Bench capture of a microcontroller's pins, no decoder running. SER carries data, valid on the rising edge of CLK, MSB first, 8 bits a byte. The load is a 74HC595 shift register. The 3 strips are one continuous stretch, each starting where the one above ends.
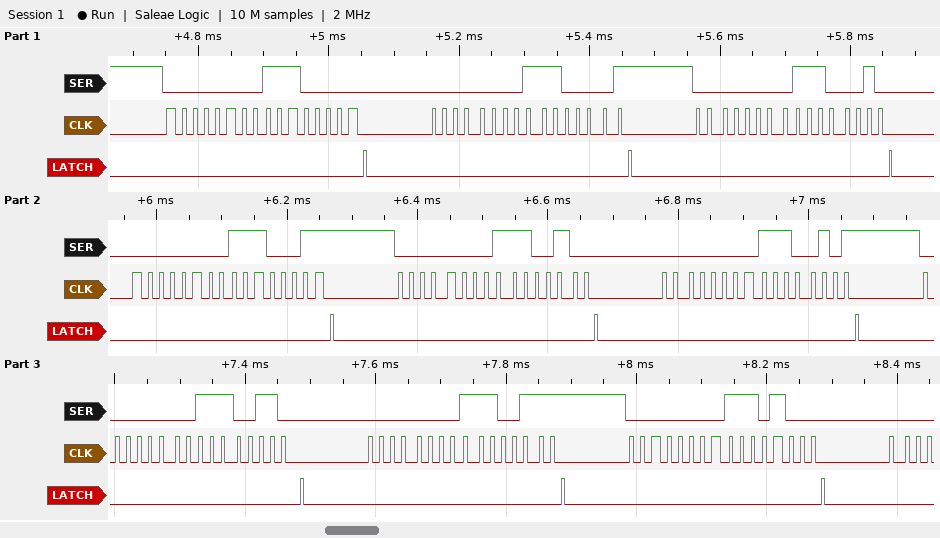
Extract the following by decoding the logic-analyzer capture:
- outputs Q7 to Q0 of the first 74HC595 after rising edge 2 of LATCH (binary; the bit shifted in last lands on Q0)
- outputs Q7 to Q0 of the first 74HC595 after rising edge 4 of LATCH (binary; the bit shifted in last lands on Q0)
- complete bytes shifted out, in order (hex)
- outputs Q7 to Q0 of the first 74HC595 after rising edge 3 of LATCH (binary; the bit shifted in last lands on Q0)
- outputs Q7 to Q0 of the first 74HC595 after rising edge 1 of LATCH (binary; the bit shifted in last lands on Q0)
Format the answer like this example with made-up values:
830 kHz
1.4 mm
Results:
11100001
11100011
00 E0 00 E1 00 E2 00 E3 00 E4 00 E5 00 E6 00 E7 00 E8
11100010
11100000
